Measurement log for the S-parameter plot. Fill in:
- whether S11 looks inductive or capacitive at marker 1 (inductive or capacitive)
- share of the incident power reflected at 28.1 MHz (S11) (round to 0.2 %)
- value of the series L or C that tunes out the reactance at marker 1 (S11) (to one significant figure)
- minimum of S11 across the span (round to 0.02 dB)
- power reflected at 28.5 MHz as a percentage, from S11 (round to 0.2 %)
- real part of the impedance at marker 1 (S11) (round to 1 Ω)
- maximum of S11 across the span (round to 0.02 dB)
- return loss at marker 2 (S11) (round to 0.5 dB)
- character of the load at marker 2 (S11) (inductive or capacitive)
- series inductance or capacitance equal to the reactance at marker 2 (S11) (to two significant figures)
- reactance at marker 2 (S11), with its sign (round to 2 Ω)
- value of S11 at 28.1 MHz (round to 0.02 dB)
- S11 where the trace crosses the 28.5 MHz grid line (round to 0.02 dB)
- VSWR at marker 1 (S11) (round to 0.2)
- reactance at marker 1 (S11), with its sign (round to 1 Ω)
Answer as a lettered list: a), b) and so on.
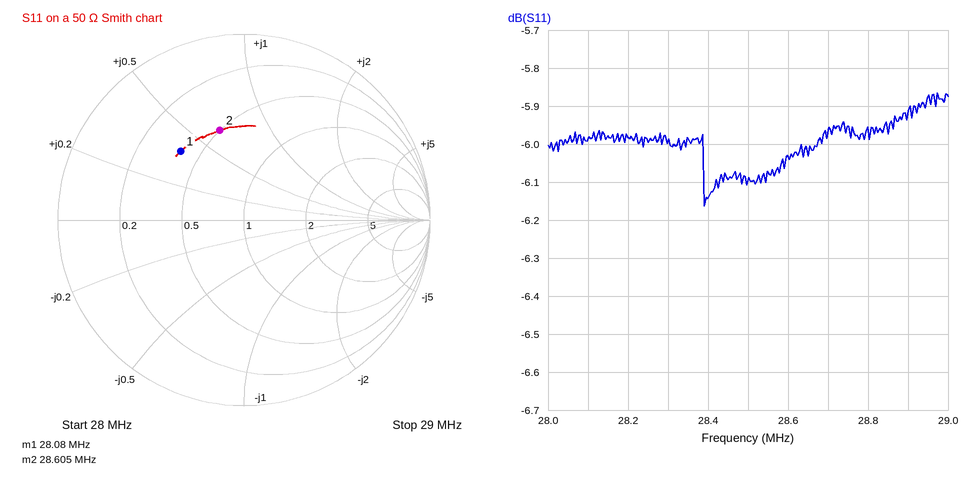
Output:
a) inductive
b) 25.2 %
c) 300 pF
d) -6.16 dB
e) 24.6 %
f) 19 Ω
g) -5.86 dB
h) 6.0 dB
i) inductive
j) 180 nH
k) +32 Ω
l) -5.98 dB
m) -6.10 dB
n) 3.0
o) +19 Ω
